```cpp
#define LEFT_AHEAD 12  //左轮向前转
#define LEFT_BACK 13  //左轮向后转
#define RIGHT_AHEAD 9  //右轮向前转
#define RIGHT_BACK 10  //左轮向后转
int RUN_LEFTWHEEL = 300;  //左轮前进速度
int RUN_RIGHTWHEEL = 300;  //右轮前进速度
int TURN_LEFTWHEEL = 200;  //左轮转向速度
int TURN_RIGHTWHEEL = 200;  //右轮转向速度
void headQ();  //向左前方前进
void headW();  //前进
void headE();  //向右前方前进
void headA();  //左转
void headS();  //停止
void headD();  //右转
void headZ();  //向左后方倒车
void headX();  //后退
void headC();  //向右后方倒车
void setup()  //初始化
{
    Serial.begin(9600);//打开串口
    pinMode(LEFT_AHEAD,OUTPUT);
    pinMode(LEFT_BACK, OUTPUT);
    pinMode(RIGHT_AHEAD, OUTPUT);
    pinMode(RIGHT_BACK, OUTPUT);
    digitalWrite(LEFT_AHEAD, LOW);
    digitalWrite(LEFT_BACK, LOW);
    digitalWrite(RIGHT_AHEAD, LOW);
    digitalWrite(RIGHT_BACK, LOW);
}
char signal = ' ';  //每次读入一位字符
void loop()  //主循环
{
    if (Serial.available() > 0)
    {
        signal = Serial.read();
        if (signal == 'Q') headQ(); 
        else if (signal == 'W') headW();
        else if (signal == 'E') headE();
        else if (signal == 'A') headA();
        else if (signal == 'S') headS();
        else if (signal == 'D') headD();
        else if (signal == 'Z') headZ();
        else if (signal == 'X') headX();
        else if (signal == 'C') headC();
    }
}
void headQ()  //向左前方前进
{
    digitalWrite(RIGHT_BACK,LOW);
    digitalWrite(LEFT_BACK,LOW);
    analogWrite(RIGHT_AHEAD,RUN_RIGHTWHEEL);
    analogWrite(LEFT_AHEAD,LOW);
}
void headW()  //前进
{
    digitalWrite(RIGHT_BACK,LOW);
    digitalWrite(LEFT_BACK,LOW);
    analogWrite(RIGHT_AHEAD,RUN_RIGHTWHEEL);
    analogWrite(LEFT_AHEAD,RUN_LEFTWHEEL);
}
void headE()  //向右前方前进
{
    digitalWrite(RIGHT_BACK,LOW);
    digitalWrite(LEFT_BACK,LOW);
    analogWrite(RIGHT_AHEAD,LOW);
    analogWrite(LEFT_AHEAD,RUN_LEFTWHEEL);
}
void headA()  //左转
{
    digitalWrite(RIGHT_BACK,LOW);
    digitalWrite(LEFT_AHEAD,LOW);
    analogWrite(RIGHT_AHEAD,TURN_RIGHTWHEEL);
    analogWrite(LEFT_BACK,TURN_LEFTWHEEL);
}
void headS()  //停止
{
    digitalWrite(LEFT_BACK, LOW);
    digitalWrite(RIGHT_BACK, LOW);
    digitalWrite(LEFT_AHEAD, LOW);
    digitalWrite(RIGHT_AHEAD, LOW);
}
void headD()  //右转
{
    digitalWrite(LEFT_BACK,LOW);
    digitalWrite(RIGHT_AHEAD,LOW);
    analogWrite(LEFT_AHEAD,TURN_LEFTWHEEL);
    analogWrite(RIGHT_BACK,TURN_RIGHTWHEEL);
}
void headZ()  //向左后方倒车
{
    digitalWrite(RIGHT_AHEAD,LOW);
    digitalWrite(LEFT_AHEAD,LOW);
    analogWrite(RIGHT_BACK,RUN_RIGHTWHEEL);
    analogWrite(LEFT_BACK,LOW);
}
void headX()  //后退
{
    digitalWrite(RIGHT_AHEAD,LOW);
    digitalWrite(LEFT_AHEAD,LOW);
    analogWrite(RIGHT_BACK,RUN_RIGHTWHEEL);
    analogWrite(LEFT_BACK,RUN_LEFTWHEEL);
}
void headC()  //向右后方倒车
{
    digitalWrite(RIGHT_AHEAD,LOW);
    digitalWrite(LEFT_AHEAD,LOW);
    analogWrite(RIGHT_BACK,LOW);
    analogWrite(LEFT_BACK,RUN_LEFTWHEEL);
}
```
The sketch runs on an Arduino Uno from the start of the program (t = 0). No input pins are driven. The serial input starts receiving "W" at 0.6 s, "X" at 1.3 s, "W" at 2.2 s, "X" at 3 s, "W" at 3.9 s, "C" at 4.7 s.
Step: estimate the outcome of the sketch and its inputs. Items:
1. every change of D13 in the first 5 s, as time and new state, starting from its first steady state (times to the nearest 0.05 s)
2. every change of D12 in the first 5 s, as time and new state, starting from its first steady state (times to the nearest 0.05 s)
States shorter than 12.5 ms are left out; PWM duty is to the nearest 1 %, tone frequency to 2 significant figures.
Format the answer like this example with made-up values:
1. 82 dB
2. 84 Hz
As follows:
1. 0 s low; 1.3 s high; 2.2 s low; 3 s high; 3.9 s low; 4.7 s high
2. 0 s low; 0.6 s high; 1.3 s low; 2.2 s high; 3 s low; 3.9 s high; 4.7 s low
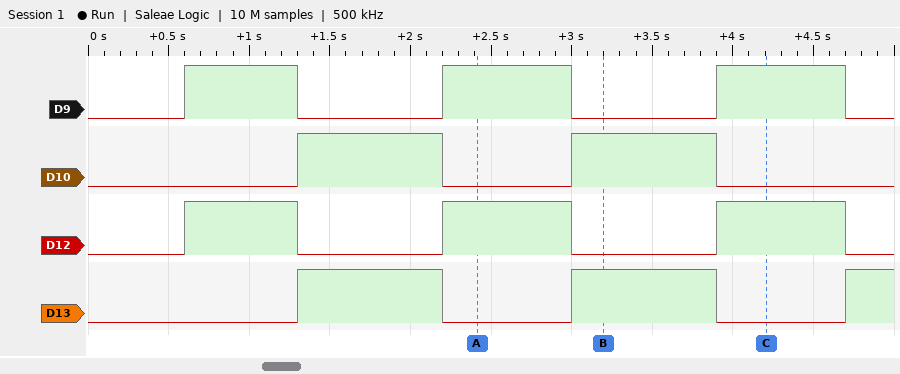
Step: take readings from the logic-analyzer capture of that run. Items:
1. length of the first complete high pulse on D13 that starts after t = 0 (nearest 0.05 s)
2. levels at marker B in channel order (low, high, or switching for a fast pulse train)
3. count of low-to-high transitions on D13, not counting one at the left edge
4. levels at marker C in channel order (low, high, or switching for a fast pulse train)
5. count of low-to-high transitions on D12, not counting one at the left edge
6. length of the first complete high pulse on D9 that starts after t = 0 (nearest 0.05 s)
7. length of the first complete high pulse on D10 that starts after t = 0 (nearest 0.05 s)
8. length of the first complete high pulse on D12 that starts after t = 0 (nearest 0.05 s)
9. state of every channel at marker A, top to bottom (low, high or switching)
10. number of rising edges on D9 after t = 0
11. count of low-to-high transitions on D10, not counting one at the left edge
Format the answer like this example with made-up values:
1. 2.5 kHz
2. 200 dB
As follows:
1. 0.90 s
2. D9 low, D10 high, D12 low, D13 high
3. 3
4. D9 high, D10 low, D12 high, D13 low
5. 3
6. 0.70 s
7. 0.90 s
8. 0.70 s
9. D9 high, D10 low, D12 high, D13 low
10. 3
11. 2
